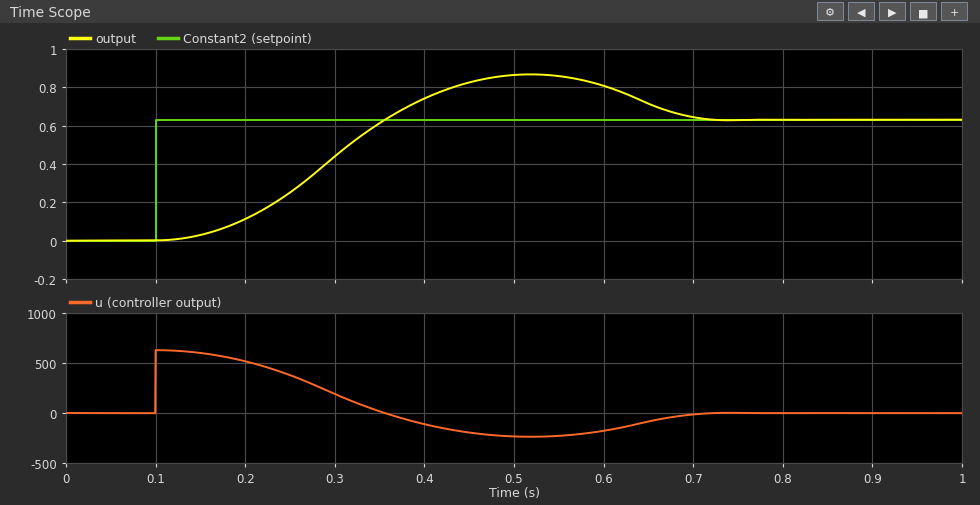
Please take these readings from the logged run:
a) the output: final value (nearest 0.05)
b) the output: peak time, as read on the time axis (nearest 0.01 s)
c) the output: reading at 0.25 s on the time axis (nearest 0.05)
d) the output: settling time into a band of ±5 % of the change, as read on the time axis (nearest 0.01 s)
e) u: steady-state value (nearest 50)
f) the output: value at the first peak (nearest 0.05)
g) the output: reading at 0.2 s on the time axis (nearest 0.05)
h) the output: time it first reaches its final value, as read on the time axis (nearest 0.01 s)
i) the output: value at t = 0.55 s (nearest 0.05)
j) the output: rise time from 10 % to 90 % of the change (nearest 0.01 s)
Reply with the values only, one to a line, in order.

0.65
0.52 s
0.25
0.68 s
0
0.85
0.10
0.36 s
0.85
0.16 s
